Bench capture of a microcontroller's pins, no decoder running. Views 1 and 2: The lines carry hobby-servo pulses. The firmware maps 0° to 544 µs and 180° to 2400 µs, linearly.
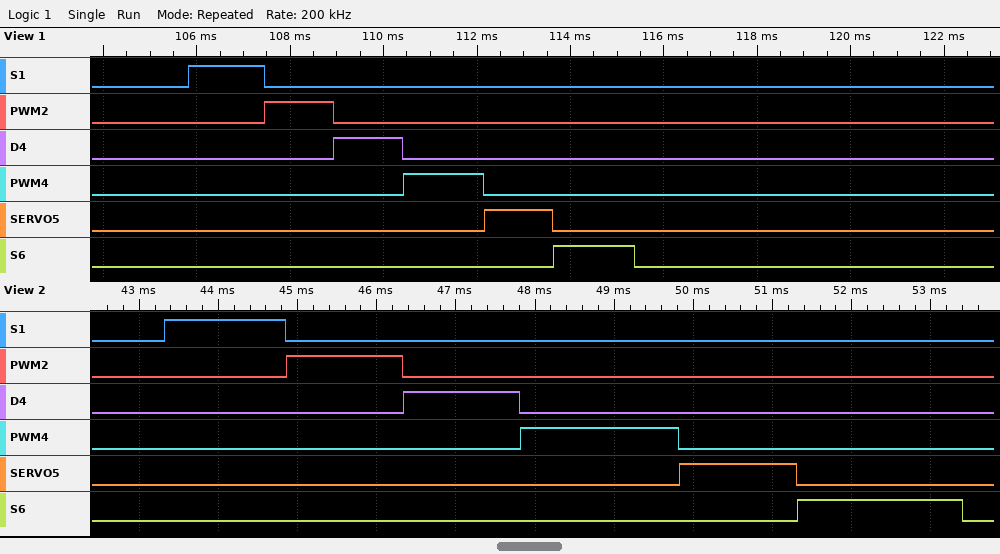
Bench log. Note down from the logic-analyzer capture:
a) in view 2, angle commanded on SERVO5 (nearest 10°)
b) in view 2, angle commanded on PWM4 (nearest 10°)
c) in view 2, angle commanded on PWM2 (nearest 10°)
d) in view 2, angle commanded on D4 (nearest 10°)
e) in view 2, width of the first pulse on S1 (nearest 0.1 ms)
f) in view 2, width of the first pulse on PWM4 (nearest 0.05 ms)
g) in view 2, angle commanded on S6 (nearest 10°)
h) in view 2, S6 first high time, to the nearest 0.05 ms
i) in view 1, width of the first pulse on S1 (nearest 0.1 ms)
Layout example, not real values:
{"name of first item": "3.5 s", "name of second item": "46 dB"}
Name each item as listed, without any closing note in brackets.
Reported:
{"in view 2, angle commanded on SERVO5": "90°", "in view 2, angle commanded on PWM4": "140°", "in view 2, angle commanded on PWM2": "90°", "in view 2, angle commanded on D4": "90°", "in view 2, width of the first pulse on S1": "1.5 ms", "in view 2, width of the first pulse on PWM4": "2.00 ms", "in view 2, angle commanded on S6": "150°", "in view 2, S6 first high time, to the nearest 0.05 ms": "2.10 ms", "in view 1, width of the first pulse on S1": "1.6 ms"}
